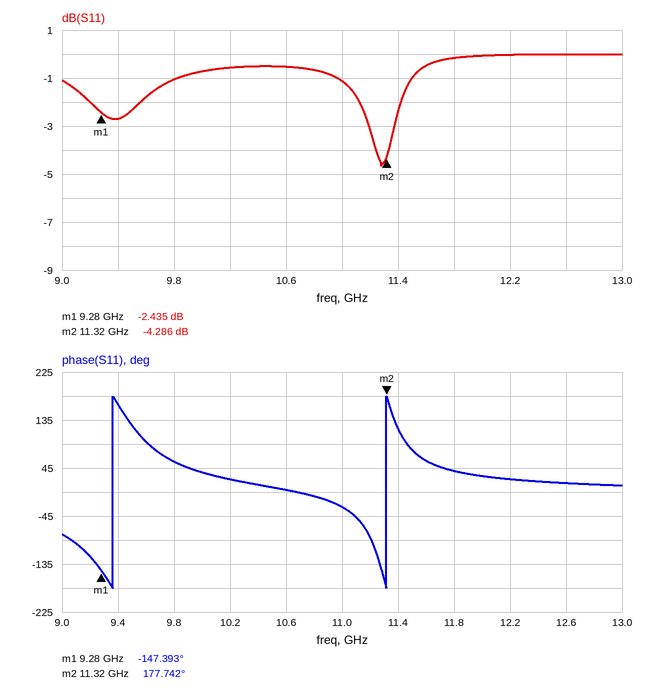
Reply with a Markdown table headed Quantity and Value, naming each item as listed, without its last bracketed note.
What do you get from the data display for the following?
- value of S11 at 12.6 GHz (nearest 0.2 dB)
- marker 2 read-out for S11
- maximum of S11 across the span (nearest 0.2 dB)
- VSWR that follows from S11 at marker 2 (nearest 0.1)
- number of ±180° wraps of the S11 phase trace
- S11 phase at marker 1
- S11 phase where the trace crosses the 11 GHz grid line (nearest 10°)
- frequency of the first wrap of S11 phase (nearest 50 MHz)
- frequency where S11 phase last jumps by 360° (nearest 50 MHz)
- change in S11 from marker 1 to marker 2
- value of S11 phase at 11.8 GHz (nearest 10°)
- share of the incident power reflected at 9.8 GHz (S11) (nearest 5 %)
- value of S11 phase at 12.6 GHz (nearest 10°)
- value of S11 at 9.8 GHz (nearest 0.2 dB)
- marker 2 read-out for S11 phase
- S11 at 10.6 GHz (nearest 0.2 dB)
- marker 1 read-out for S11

| Quantity | Value |
|---|---|
| value of S11 at 12.6 GHz | 0.0 dB |
| marker 2 read-out for S11 | -4.286 dB |
| maximum of S11 across the span | 0.0 dB |
| VSWR that follows from S11 at marker 2 | 4.1 |
| number of ±180° wraps of the S11 phase trace | 2 |
| S11 phase at marker 1 | -147.393° |
| S11 phase where the trace crosses the 11 GHz grid line | -30° |
| frequency of the first wrap of S11 phase | 9.35 GHz |
| frequency where S11 phase last jumps by 360° | 11.30 GHz |
| change in S11 from marker 1 to marker 2 | -1.851 dB |
| value of S11 phase at 11.8 GHz | 40° |
| share of the incident power reflected at 9.8 GHz (S11) | 80 % |
| value of S11 phase at 12.6 GHz | 20° |
| value of S11 at 9.8 GHz | -1.0 dB |
| marker 2 read-out for S11 phase | 177.742° |
| S11 at 10.6 GHz | -0.6 dB |
| marker 1 read-out for S11 | -2.435 dB |
